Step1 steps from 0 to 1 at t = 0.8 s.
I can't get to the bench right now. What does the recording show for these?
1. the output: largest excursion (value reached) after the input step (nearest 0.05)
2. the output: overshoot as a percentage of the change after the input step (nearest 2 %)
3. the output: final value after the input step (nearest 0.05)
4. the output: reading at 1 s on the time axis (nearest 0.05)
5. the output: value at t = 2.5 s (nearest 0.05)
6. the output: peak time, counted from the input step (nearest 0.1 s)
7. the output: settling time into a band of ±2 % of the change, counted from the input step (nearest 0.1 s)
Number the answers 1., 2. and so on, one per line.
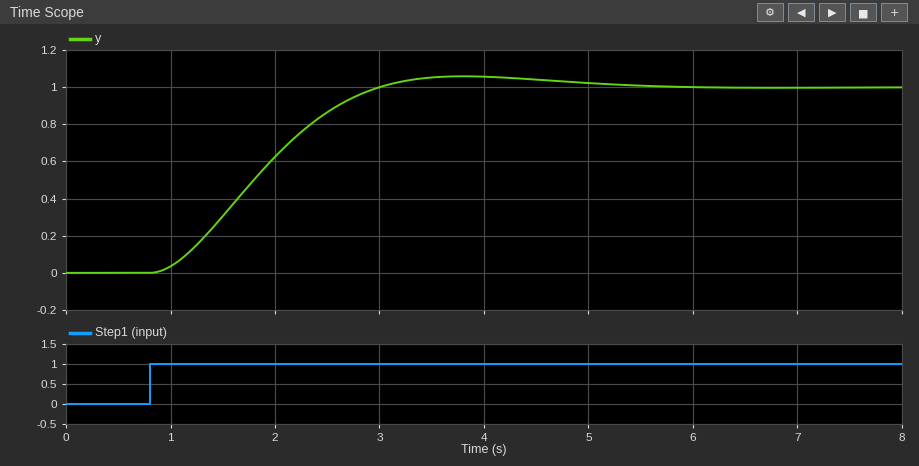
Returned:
1. 1.05
2. 6 %
3. 1.00
4. 0.05
5. 0.85
6. 3.0 s
7. 4.3 s
